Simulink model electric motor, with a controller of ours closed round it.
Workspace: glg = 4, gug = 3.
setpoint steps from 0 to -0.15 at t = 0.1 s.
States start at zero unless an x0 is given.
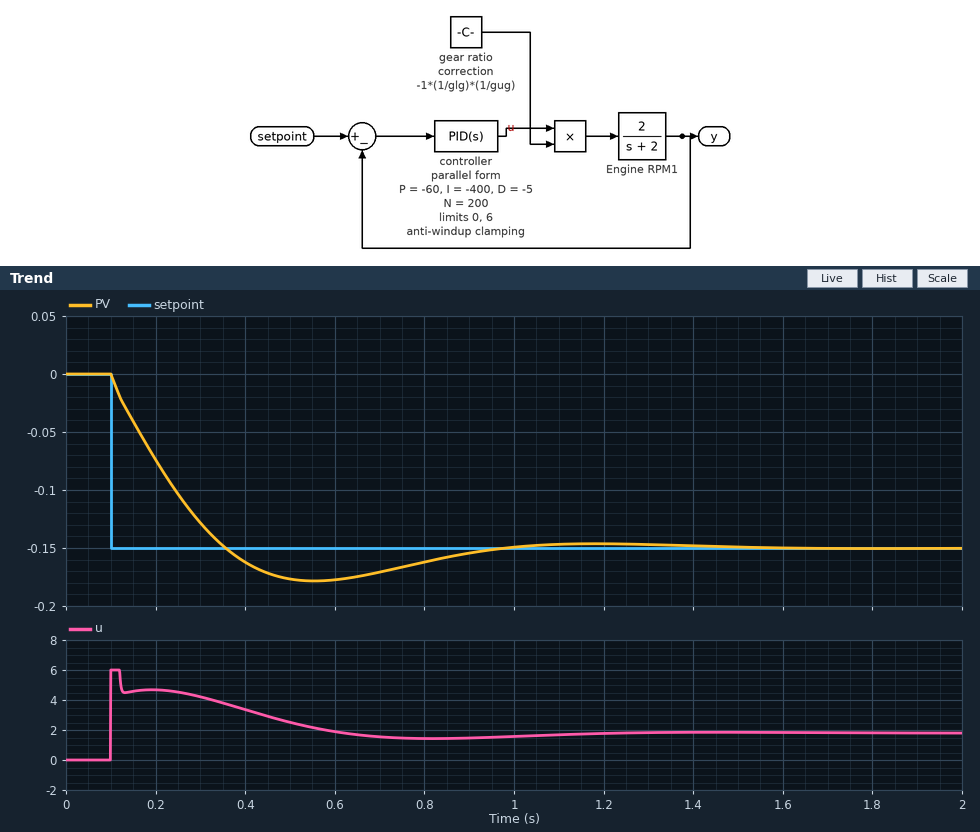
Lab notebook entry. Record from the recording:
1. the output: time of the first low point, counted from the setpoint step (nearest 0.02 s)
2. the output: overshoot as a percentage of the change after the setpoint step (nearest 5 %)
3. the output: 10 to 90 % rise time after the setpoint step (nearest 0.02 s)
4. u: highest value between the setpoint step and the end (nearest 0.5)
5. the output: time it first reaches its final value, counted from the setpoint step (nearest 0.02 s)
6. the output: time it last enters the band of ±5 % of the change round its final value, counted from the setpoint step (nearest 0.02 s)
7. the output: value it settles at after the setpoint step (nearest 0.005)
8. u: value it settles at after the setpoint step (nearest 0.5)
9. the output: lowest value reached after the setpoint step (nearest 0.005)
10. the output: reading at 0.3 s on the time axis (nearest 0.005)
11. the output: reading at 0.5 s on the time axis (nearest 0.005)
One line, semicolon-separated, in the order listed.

0.46 s; 20 %; 0.20 s; 6.0; 0.26 s; 0.76 s; -0.150; 2.0; -0.180; -0.130; -0.175
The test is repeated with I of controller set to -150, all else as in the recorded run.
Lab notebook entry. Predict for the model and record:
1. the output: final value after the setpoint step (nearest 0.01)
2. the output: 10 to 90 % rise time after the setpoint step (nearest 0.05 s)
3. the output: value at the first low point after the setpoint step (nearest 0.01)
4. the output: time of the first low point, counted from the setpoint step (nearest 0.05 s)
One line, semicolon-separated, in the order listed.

-0.15; 0.30 s; -0.16; 0.70 s
